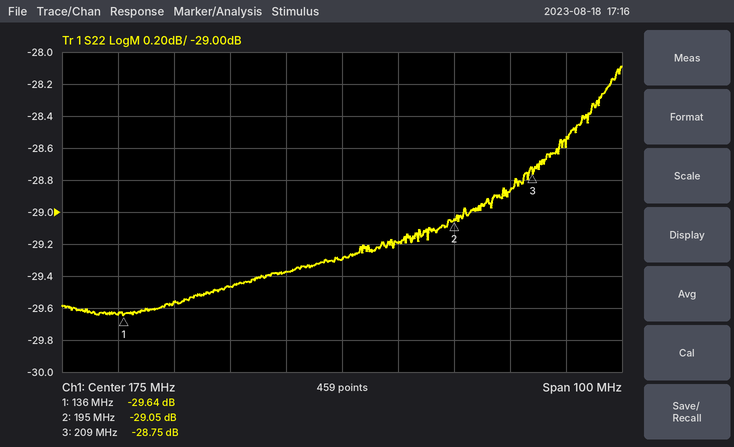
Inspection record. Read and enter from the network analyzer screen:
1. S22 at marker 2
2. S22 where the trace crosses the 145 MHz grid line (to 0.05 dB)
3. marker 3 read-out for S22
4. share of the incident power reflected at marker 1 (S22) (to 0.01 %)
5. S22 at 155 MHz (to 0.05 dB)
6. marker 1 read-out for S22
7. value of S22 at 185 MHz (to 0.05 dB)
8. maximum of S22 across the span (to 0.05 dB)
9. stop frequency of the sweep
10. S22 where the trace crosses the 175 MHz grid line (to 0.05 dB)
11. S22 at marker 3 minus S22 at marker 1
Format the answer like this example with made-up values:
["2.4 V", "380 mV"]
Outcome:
["-29.05 dB", "-29.55 dB", "-28.75 dB", "0.11 %", "-29.45 dB", "-29.64 dB", "-29.20 dB", "-28.10 dB", "225 MHz", "-29.30 dB", "0.89 dB"]
